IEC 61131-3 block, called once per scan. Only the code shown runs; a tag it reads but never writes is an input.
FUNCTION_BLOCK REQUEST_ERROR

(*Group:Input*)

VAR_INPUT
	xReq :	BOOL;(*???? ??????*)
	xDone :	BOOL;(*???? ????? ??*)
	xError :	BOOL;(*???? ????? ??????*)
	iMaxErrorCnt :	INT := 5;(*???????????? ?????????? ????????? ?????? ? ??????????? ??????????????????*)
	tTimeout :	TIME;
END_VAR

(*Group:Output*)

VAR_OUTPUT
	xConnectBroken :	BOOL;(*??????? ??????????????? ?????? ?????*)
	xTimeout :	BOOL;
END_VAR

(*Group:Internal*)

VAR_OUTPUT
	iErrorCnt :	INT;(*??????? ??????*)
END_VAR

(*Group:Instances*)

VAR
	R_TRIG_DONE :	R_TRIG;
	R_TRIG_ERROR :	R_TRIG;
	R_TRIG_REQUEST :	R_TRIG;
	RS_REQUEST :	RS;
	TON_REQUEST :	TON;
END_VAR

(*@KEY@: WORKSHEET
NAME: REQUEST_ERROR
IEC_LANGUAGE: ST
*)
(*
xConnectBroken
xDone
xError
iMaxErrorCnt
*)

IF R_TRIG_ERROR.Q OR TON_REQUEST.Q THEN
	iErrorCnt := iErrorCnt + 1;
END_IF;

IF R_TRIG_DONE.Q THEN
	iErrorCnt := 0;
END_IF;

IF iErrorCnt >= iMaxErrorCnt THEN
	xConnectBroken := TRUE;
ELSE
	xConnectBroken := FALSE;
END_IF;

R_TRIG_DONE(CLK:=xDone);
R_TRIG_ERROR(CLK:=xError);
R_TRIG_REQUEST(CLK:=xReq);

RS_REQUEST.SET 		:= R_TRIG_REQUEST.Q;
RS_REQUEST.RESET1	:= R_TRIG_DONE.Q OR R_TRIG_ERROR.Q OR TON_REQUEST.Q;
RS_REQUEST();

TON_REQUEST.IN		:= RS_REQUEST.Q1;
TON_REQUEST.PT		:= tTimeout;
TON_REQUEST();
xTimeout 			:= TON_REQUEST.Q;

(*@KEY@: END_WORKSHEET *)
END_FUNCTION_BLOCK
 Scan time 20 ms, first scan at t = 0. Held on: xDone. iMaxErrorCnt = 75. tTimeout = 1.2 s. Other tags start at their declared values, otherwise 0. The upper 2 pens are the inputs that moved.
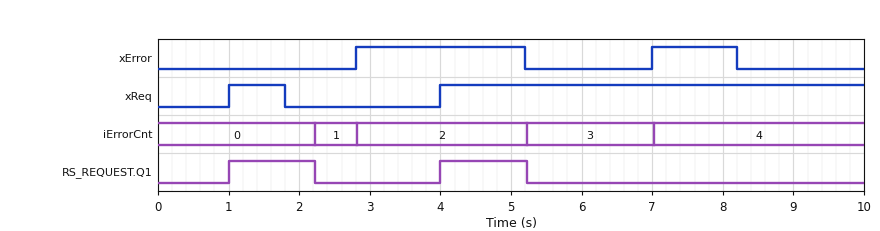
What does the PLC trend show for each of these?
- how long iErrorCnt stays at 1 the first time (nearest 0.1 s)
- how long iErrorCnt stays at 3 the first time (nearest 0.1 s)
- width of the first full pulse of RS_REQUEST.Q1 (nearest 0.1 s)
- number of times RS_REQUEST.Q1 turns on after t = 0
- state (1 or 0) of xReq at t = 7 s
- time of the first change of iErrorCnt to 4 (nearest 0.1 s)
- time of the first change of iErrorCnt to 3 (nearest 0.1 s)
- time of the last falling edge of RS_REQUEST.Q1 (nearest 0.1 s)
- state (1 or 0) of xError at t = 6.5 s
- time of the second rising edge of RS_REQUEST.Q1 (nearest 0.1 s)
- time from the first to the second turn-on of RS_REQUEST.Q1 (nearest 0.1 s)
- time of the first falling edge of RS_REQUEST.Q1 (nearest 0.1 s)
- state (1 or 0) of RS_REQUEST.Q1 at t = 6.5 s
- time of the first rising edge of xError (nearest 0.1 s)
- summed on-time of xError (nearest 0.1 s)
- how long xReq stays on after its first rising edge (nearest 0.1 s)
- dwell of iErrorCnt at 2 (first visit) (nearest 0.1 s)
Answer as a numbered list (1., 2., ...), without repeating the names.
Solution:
1. 0.6 s
2. 1.8 s
3. 1.2 s
4. 2
5. 1
6. 7.0 s
7. 5.2 s
8. 5.2 s
9. 0
10. 4.0 s
11. 3.0 s
12. 2.2 s
13. 0
14. 2.8 s
15. 3.6 s
16. 0.8 s
17. 2.4 s
